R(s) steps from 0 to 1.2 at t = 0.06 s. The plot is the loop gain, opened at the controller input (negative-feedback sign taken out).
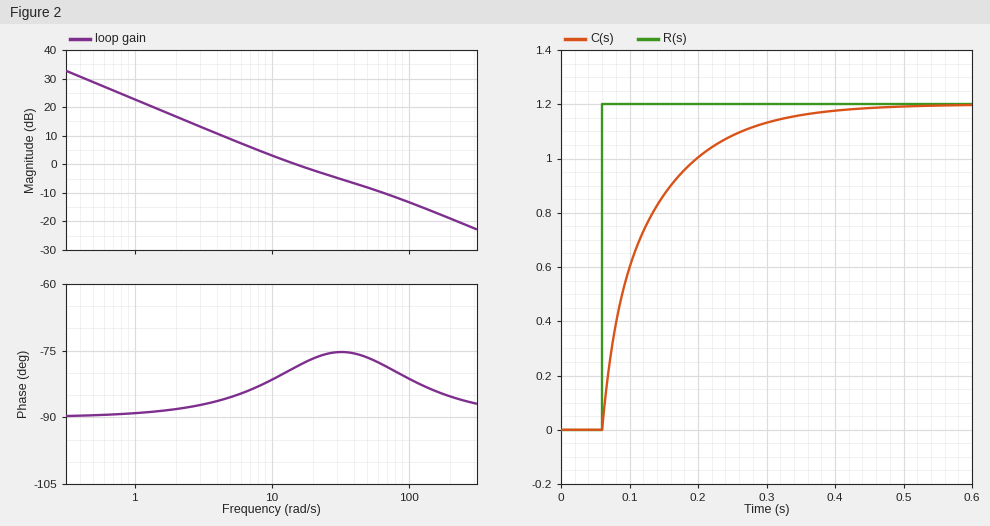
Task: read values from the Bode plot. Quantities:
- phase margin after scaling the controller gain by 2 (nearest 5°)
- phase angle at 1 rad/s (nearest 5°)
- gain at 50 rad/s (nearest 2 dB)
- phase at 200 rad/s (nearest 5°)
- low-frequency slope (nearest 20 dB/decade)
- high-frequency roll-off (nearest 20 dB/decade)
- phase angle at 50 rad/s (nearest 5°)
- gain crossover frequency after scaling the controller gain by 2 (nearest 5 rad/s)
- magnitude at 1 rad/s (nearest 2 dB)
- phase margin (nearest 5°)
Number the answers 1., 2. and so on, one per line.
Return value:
1. 105°
2. -90°
3. -8 dB
4. -85°
5. -20 dB/decade
6. -20 dB/decade
7. -75°
8. 35 rad/s
9. 22 dB
10. 100°
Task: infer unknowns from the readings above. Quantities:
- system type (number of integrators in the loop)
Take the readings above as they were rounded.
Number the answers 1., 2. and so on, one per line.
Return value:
1. 1
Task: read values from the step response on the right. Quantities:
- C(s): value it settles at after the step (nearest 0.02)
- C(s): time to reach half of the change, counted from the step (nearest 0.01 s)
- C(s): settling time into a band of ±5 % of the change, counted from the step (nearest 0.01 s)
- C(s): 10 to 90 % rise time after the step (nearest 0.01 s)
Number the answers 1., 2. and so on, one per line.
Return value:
1. 1.20
2. 0.04 s
3. 0.25 s
4. 0.18 s
